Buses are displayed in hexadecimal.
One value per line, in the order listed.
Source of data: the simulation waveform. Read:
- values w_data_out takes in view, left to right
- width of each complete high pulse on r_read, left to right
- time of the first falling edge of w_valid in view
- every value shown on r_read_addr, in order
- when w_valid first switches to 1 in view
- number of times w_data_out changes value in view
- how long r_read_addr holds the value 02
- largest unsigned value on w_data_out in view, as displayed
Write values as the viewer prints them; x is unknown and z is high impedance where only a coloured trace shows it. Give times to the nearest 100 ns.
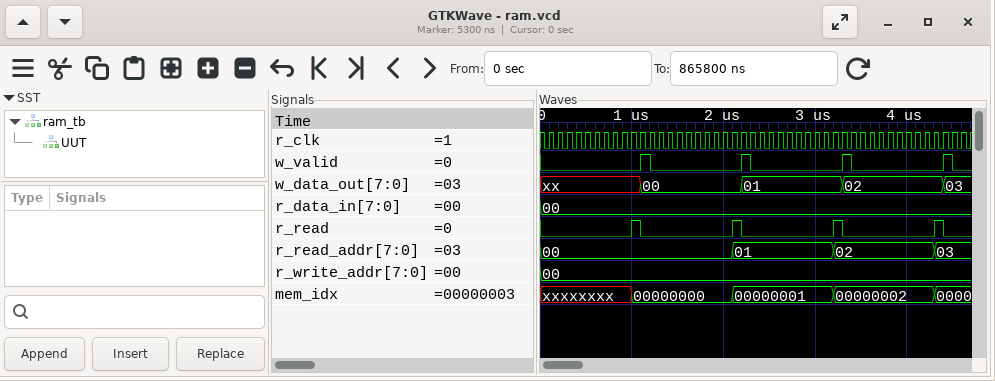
xx, 00, 01, 02, 03
100 ns, 100 ns, 100 ns, 100 ns
1200 ns
00, 01, 02, 03
1100 ns
4
1100 ns
03
